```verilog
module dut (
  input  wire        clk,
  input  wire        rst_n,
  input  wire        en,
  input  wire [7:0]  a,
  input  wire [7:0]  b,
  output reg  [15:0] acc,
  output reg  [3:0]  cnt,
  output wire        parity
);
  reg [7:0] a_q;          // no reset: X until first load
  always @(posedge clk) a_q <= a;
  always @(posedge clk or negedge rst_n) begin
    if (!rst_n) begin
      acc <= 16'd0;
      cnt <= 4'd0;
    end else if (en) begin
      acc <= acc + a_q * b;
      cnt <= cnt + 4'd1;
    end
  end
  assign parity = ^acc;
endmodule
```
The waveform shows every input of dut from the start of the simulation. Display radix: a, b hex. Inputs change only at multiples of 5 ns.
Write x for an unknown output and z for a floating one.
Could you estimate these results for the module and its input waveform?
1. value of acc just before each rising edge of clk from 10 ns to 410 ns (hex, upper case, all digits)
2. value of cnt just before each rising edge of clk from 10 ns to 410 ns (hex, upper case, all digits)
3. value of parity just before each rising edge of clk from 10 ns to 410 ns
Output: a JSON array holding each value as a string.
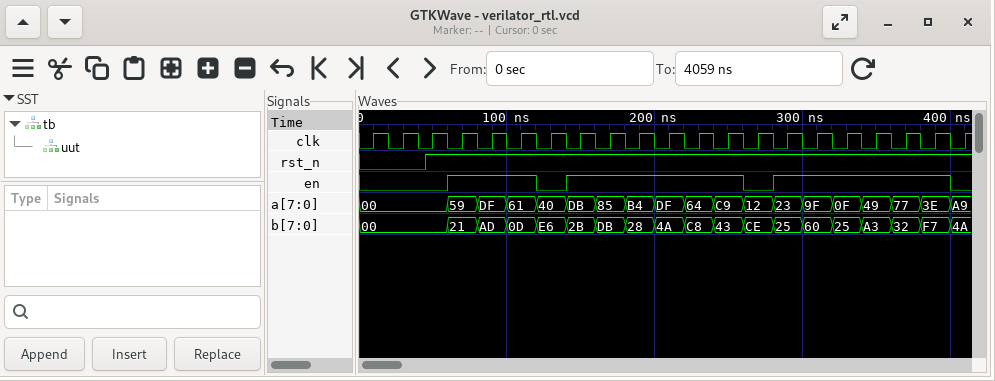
["0000, 0000, 0000, 0000, 0000, 3C25, 4778, 4778, 5238, 0D91, 2259, 5661, 0499, 1EC5, 1EC5, 215F, 2E7F, 457A, 4F07, 5D49, D01A", "0, 0, 0, 0, 1, 2, 3, 3, 4, 5, 6, 7, 8, 9, 9, A, B, C, D, E, F", "0 0 0 0 0 1 0 0 0 0 0 1 1 0 0 0 1 0 0 0 0"]
